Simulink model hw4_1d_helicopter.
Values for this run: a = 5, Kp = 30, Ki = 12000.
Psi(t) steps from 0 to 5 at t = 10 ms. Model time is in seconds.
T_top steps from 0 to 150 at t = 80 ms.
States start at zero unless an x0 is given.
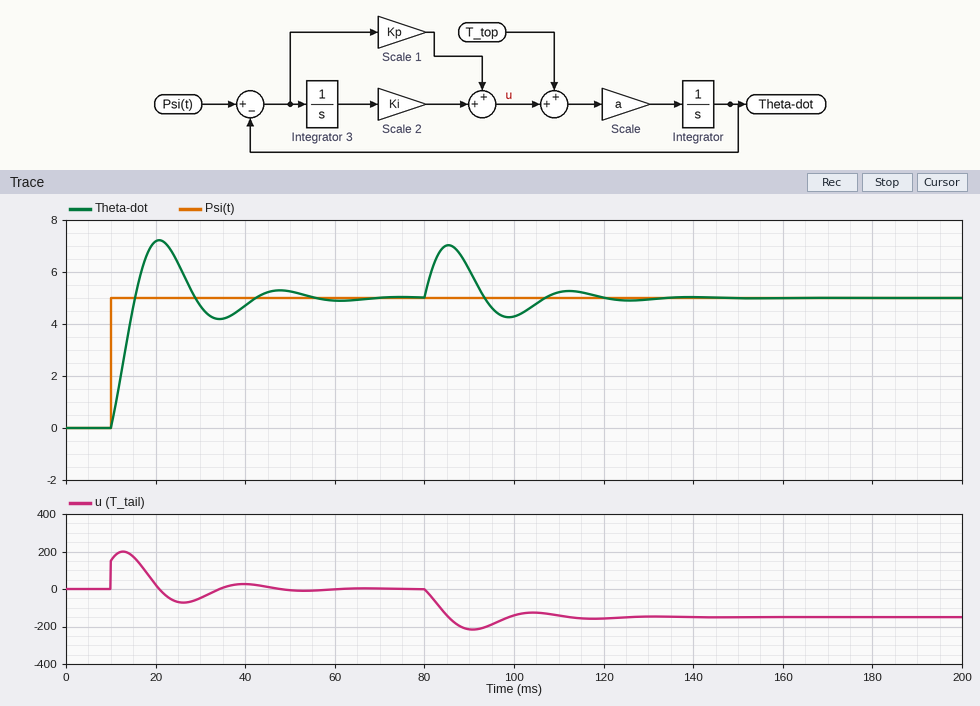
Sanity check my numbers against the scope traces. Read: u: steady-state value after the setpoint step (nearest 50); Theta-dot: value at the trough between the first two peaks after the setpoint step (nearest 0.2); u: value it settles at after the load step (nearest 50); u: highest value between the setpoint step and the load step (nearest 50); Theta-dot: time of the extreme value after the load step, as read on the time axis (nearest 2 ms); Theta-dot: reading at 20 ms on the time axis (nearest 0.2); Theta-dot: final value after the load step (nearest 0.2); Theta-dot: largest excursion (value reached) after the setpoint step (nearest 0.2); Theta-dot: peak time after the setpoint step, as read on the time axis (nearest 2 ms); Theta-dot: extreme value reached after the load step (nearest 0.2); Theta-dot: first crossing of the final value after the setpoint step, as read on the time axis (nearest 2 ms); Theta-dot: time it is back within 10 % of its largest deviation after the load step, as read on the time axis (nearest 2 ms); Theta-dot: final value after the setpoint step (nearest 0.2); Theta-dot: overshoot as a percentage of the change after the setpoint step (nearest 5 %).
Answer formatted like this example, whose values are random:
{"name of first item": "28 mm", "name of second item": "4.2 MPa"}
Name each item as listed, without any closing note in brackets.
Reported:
{"u: steady-state value after the setpoint step": "0", "Theta-dot: value at the trough between the first two peaks after the setpoint step": "4.2", "u: value it settles at after the load step": "-150", "u: highest value between the setpoint step and the load step": "200", "Theta-dot: time of the extreme value after the load step, as read on the time axis": "86 ms", "Theta-dot: reading at 20 ms on the time axis": "7.2", "Theta-dot: final value after the load step": "5.0", "Theta-dot: largest excursion (value reached) after the setpoint step": "7.2", "Theta-dot: peak time after the setpoint step, as read on the time axis": "20 ms", "Theta-dot: extreme value reached after the load step": "7.0", "Theta-dot: first crossing of the final value after the setpoint step, as read on the time axis": "16 ms", "Theta-dot: time it is back within 10 % of its largest deviation after the load step, as read on the time axis": "116 ms", "Theta-dot: final value after the setpoint step": "5.0", "Theta-dot: overshoot as a percentage of the change after the setpoint step": "45 %"}
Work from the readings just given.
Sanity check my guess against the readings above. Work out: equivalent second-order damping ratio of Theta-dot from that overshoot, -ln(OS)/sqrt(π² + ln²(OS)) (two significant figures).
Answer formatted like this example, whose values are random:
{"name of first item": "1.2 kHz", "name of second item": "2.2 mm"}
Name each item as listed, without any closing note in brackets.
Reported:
{"equivalent second-order damping ratio of Theta-dot from that overshoot, -ln(OS)/sqrt(π² + ln²(OS))": "0.25"}
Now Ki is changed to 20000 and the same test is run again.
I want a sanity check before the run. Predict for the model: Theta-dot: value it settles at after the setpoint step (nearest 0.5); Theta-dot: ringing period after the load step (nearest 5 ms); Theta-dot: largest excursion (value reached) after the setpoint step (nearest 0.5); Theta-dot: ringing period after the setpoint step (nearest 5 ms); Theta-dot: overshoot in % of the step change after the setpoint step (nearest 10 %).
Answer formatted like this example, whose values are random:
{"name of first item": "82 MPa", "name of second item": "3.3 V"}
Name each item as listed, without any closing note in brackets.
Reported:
{"Theta-dot: value it settles at after the setpoint step": "5.0", "Theta-dot: ringing period after the load step": "20 ms", "Theta-dot: largest excursion (value reached) after the setpoint step": "7.5", "Theta-dot: ringing period after the setpoint step": "20 ms", "Theta-dot: overshoot in % of the step change after the setpoint step": "50 %"}
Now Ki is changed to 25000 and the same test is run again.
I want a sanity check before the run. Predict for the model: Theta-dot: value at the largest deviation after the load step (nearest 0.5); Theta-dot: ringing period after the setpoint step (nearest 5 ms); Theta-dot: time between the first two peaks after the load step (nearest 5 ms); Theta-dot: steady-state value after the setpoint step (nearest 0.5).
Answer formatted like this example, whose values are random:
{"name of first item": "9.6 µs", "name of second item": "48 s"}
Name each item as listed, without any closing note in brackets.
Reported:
{"Theta-dot: value at the largest deviation after the load step": "6.5", "Theta-dot: ringing period after the setpoint step": "20 ms", "Theta-dot: time between the first two peaks after the load step": "20 ms", "Theta-dot: steady-state value after the setpoint step": "5.0"}
